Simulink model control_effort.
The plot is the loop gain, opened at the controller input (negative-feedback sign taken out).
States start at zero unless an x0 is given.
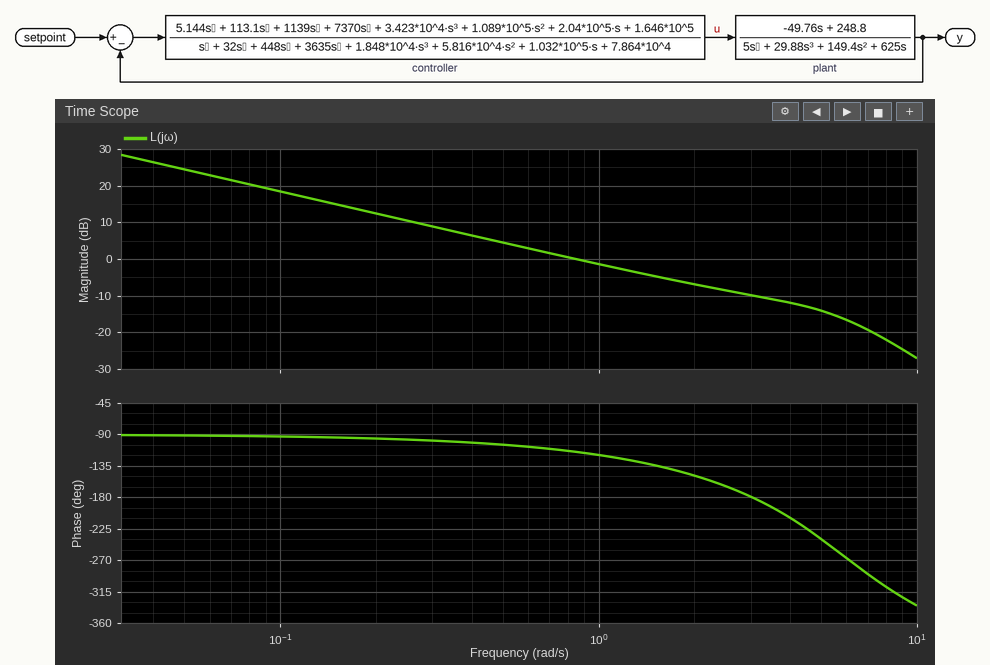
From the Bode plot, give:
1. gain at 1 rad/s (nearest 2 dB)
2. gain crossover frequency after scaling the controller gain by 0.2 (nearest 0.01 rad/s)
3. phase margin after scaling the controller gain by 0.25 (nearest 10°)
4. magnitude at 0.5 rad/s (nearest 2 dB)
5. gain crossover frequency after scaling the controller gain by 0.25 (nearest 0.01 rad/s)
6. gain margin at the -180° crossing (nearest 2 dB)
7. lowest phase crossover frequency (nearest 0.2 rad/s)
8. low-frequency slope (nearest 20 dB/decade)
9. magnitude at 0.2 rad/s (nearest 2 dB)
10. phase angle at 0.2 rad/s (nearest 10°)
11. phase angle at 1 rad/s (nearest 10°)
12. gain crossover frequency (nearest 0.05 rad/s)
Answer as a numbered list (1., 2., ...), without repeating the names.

1. -2 dB
2. 0.17 rad/s
3. 80°
4. 4 dB
5. 0.21 rad/s
6. 10 dB
7. 3.0 rad/s
8. -20 dB/decade
9. 12 dB
10. -100°
11. -120°
12. 0.85 rad/s
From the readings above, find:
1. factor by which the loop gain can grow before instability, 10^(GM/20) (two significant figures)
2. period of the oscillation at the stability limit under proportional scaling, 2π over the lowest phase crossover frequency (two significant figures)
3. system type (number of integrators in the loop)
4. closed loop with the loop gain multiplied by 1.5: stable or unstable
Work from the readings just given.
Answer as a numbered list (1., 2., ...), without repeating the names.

1. 3.2
2. 2.1 s
3. 1
4. stable
